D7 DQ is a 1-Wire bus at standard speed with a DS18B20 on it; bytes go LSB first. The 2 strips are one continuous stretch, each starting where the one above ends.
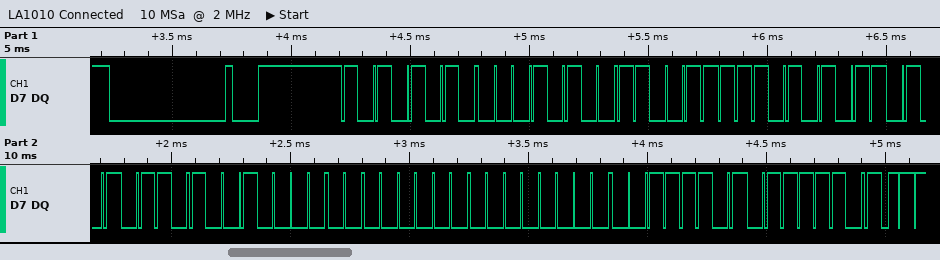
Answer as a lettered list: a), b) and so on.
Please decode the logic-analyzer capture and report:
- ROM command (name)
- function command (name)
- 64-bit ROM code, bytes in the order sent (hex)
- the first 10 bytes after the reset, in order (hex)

a) Match ROM
b) Read Scratchpad
c) 28 F3 D5 6A 09 00 00 BC
d) 55 28 F3 D5 6A 09 00 00 BC BE
